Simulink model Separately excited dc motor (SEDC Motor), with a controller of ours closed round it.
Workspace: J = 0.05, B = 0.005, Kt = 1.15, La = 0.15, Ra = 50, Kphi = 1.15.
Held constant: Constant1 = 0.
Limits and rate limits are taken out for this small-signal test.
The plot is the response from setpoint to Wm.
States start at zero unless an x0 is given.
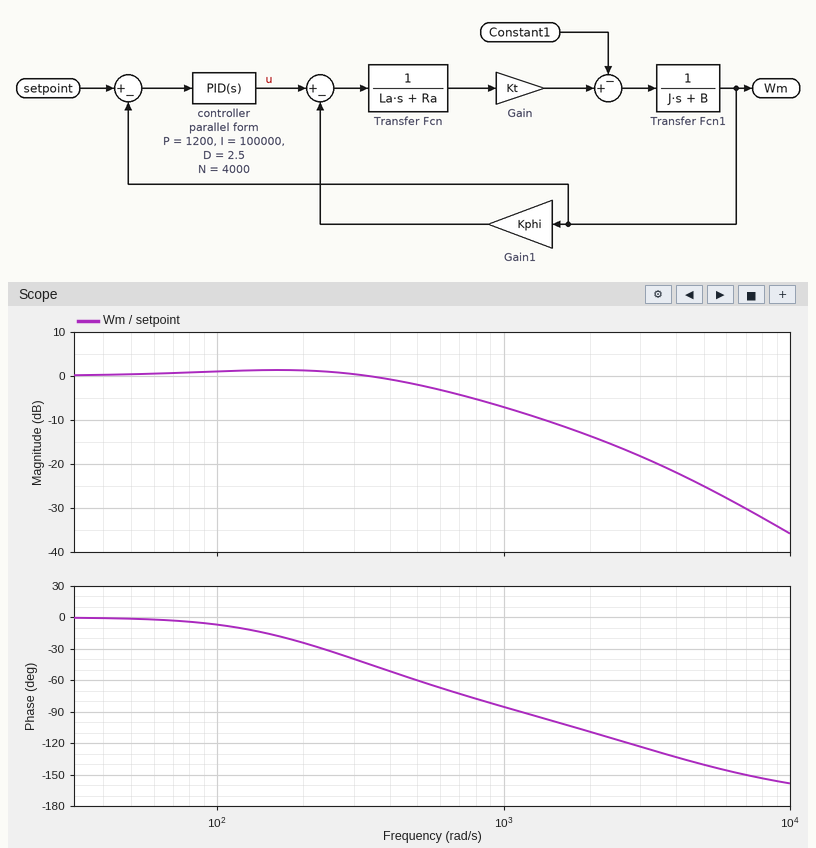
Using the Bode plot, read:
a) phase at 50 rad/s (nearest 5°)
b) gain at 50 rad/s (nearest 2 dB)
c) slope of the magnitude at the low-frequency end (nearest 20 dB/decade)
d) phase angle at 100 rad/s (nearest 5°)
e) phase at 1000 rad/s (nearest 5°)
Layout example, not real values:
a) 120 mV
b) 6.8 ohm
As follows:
a) 0°
b) 0 dB
c) 0 dB/decade
d) -5°
e) -85°
